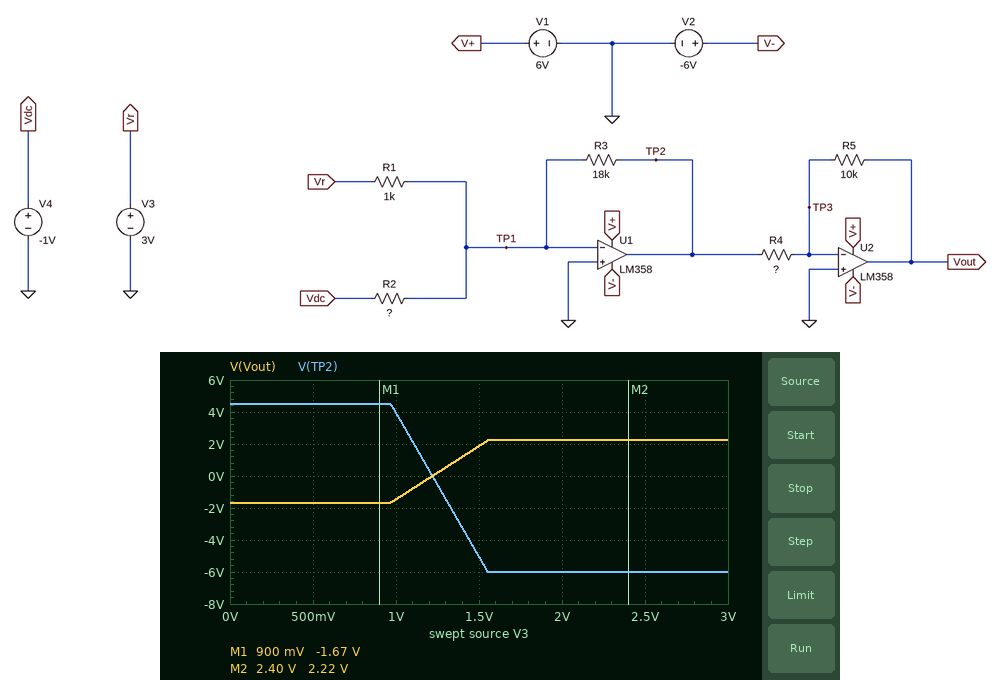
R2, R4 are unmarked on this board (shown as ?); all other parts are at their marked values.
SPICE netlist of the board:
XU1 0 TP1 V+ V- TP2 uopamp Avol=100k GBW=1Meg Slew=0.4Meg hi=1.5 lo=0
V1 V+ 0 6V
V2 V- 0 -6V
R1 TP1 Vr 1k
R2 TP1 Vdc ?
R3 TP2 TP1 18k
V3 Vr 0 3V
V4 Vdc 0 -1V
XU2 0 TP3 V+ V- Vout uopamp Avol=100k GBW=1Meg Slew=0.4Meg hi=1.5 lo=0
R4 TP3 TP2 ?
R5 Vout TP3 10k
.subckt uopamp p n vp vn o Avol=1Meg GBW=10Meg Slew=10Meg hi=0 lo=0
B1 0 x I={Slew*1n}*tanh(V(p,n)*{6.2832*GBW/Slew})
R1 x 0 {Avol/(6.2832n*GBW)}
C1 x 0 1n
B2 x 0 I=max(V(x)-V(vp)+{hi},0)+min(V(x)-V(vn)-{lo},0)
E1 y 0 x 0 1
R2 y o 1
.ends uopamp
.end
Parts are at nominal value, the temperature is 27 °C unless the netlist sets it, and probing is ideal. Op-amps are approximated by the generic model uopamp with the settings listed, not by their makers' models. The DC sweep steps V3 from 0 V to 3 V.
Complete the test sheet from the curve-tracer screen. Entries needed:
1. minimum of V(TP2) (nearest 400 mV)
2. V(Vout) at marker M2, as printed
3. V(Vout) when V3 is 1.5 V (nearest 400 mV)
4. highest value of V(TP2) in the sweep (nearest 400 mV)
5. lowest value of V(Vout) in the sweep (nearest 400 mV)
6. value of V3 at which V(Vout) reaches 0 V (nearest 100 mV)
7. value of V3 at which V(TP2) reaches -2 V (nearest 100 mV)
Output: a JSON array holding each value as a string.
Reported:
["-6.0 V", "2.22 V", "2.0 V", "4.4 V", "-1.6 V", "1.2 V", "1.3 V"]
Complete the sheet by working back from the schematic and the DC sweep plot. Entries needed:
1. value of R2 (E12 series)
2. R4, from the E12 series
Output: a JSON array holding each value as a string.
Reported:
["820 Ω", "27 kΩ"]
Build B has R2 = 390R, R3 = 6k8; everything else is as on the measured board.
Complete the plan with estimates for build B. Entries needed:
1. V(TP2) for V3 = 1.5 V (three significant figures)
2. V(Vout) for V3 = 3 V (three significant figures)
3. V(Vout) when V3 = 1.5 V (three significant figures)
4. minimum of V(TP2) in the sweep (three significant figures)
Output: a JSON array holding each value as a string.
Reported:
["4.50 V", "1.10 V", "-1.67 V", "-2.96 V"]
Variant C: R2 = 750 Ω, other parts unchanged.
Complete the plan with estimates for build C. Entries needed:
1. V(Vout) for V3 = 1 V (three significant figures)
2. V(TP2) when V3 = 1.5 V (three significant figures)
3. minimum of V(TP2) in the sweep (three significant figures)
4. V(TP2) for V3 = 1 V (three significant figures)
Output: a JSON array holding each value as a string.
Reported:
["-1.67 V", "-3.00 V", "-6.00 V", "4.50 V"]
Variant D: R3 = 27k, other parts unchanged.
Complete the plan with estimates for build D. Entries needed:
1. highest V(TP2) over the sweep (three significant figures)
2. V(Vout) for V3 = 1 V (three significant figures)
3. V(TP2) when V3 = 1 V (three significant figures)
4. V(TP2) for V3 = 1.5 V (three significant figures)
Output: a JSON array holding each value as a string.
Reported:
["4.50 V", "-1.67 V", "4.50 V", "-6.00 V"]
